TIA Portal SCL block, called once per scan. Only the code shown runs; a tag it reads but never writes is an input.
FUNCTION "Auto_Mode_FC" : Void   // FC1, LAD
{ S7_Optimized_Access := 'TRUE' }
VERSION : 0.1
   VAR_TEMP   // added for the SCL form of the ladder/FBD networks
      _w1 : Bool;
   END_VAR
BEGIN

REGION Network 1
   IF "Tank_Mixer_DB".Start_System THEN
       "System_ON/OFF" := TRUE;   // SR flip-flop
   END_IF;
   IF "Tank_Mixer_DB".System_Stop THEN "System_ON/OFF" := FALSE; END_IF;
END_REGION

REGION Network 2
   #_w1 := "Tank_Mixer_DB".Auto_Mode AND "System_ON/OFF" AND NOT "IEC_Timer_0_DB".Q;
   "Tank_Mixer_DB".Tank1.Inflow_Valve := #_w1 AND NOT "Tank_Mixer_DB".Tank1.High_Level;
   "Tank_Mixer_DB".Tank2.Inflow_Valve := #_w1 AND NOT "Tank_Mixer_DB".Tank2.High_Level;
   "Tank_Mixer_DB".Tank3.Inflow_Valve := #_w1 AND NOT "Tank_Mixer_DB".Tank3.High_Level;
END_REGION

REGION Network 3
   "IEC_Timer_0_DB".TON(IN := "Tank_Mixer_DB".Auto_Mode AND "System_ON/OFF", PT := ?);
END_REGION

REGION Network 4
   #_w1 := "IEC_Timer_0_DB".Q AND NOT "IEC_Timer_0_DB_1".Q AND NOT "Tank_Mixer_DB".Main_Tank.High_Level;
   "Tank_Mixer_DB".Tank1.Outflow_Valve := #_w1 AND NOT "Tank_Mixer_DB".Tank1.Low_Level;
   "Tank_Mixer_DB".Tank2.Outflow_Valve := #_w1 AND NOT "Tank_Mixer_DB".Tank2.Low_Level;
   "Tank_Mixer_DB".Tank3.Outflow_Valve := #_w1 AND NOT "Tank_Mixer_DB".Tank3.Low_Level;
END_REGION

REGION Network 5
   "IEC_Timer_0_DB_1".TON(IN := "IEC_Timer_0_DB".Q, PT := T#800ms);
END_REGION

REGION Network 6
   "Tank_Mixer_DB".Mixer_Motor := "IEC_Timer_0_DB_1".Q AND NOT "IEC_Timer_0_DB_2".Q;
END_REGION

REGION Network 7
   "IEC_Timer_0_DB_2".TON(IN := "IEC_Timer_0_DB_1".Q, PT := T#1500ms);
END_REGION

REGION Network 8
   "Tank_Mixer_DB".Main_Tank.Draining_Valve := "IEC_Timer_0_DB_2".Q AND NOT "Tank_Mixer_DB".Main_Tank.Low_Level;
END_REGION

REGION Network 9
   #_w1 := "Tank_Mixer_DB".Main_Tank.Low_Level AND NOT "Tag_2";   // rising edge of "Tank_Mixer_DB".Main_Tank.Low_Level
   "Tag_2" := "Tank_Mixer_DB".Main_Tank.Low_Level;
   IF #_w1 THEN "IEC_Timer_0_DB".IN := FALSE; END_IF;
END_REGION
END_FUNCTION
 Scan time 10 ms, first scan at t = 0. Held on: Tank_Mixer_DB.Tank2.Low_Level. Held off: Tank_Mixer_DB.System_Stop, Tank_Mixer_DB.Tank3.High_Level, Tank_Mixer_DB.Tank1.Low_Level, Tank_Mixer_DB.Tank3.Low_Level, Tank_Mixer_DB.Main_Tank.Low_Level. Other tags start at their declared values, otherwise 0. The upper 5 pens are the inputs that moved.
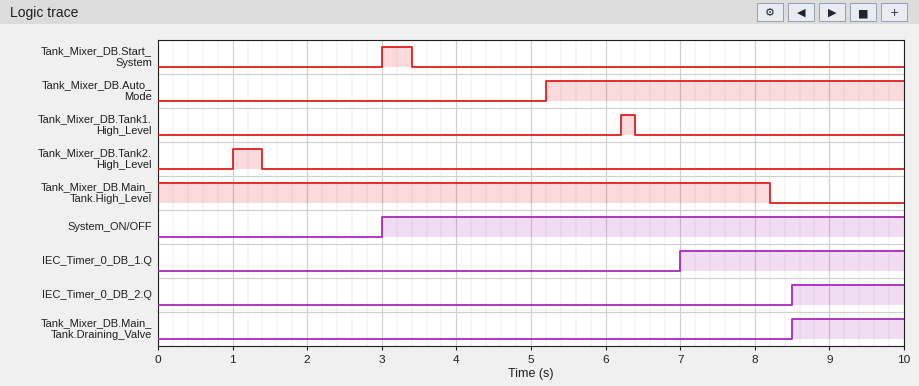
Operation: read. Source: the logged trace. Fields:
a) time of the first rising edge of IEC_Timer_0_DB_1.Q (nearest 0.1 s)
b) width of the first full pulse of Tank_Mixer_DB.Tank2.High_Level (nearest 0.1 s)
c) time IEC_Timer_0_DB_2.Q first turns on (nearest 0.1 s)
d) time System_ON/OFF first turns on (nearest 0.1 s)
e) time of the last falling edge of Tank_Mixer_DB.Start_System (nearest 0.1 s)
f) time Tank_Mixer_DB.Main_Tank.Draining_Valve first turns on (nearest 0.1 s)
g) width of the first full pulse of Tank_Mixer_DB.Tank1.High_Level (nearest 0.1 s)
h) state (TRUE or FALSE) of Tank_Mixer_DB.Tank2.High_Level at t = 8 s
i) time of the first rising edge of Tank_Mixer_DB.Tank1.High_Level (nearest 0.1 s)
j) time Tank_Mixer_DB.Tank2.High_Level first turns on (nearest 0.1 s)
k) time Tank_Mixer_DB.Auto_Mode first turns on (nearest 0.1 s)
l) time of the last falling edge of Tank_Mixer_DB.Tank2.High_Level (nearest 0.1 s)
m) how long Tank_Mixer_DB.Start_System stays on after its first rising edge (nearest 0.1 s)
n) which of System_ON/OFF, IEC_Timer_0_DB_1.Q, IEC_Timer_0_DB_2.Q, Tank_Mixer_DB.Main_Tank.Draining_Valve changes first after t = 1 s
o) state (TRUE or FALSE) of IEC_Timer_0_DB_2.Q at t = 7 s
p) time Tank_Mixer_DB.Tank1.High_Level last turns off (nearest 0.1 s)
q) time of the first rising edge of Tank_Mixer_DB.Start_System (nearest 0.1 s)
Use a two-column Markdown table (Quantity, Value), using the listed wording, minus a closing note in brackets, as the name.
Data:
| Quantity | Value |
|---|---|
| time of the first rising edge of IEC_Timer_0_DB_1.Q | 7.0 s |
| width of the first full pulse of Tank_Mixer_DB.Tank2.High_Level | 0.4 s |
| time IEC_Timer_0_DB_2.Q first turns on | 8.5 s |
| time System_ON/OFF first turns on | 3.0 s |
| time of the last falling edge of Tank_Mixer_DB.Start_System | 3.4 s |
| time Tank_Mixer_DB.Main_Tank.Draining_Valve first turns on | 8.5 s |
| width of the first full pulse of Tank_Mixer_DB.Tank1.High_Level | 0.2 s |
| state (TRUE or FALSE) of Tank_Mixer_DB.Tank2.High_Level at t = 8 s | FALSE |
| time of the first rising edge of Tank_Mixer_DB.Tank1.High_Level | 6.2 s |
| time Tank_Mixer_DB.Tank2.High_Level first turns on | 1.0 s |
| time Tank_Mixer_DB.Auto_Mode first turns on | 5.2 s |
| time of the last falling edge of Tank_Mixer_DB.Tank2.High_Level | 1.4 s |
| how long Tank_Mixer_DB.Start_System stays on after its first rising edge | 0.4 s |
| which of System_ON/OFF, IEC_Timer_0_DB_1.Q, IEC_Timer_0_DB_2.Q, Tank_Mixer_DB.Main_Tank.Draining_Valve changes first after t = 1 s | System_ON/OFF |
| state (TRUE or FALSE) of IEC_Timer_0_DB_2.Q at t = 7 s | FALSE |
| time Tank_Mixer_DB.Tank1.High_Level last turns off | 6.4 s |
| time of the first rising edge of Tank_Mixer_DB.Start_System | 3.0 s |
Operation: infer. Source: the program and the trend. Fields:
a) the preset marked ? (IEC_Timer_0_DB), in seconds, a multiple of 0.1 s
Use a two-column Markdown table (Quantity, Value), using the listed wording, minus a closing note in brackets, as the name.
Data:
| Quantity | Value |
|---|---|
| the preset marked ? (IEC_Timer_0_DB), in seconds, a multiple of 0.1 s | 1.0 s |
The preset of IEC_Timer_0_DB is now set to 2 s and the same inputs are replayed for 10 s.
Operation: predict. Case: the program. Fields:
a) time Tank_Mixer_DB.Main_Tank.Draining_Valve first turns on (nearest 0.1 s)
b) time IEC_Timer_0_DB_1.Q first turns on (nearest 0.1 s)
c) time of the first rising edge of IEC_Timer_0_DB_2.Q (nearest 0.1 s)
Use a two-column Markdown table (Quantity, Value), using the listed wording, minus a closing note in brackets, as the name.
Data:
| Quantity | Value |
|---|---|
| time Tank_Mixer_DB.Main_Tank.Draining_Valve first turns on | 9.5 s |
| time IEC_Timer_0_DB_1.Q first turns on | 8.0 s |
| time of the first rising edge of IEC_Timer_0_DB_2.Q | 9.5 s |
